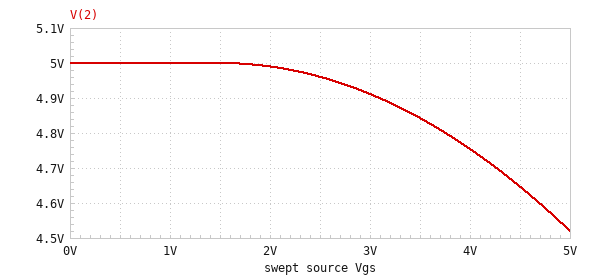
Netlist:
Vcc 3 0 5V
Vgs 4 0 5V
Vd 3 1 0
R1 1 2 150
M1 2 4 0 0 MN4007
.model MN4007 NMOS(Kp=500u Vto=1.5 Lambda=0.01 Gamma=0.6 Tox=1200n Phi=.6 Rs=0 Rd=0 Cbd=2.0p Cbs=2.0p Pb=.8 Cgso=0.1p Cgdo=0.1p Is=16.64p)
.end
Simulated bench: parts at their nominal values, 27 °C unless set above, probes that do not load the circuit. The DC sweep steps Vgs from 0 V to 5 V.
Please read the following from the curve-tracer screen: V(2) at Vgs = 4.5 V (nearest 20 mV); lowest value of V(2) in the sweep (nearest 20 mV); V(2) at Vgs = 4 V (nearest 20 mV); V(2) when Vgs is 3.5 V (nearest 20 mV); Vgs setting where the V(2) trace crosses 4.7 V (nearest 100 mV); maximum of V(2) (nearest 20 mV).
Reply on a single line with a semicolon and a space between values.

4.64 V; 4.52 V; 4.76 V; 4.84 V; 4.3 V; 5.00 V
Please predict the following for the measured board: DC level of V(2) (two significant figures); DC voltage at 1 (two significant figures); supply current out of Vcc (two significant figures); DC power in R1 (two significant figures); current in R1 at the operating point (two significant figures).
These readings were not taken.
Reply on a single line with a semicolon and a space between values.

4.5 V; 5.0 V; 3.2 mA; 1.5 mW; 3.2 mA
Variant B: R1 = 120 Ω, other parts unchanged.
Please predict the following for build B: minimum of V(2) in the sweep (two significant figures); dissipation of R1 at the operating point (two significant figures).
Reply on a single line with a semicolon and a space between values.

4.6 V; 1.2 mW
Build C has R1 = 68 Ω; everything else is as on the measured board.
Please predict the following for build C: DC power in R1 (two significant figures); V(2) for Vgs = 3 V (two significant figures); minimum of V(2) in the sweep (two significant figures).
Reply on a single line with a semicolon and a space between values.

700 µW; 5.0 V; 4.8 V
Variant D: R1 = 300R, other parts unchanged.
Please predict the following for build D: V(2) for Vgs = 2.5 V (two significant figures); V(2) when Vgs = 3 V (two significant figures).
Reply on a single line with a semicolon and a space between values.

4.9 V; 4.8 V
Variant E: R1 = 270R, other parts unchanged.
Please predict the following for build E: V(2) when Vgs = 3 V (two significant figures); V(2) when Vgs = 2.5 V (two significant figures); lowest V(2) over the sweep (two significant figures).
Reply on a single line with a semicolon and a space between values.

4.8 V; 4.9 V; 4.1 V
